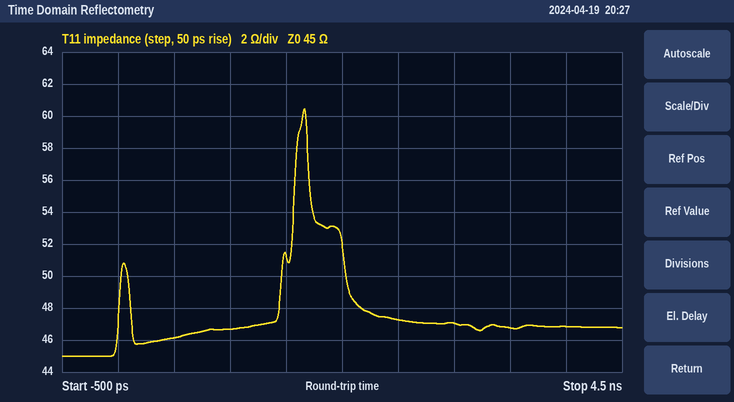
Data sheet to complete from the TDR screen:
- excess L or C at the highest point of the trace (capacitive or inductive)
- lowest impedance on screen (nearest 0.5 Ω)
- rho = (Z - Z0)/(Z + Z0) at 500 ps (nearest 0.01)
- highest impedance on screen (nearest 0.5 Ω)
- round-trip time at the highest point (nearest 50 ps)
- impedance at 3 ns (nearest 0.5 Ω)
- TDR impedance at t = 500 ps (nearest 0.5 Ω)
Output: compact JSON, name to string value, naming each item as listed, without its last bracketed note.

{"excess L or C at the highest point of the trace": "inductive", "lowest impedance on screen": "45.0 Ω", "rho = (Z - Z0)/(Z + Z0) at 500 ps": "+0.01", "highest impedance on screen": "60.5 Ω", "round-trip time at the highest point": "1.65 ns", "impedance at 3 ns": "47.0 Ω", "TDR impedance at t = 500 ps": "46.0 Ω"}
